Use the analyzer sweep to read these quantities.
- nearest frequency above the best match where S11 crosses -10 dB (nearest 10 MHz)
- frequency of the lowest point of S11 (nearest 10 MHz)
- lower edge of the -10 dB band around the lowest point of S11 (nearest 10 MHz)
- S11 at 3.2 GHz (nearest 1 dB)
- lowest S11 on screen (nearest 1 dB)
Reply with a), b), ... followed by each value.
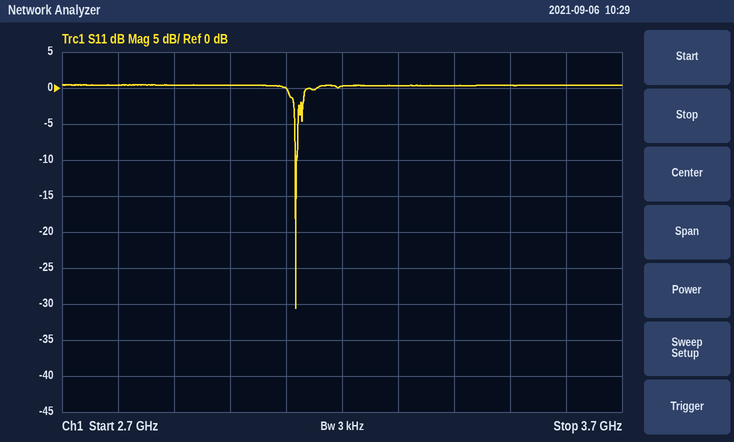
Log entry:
a) 3.12 GHz
b) 3.12 GHz
c) 3.12 GHz
d) 0 dB
e) -31 dB
